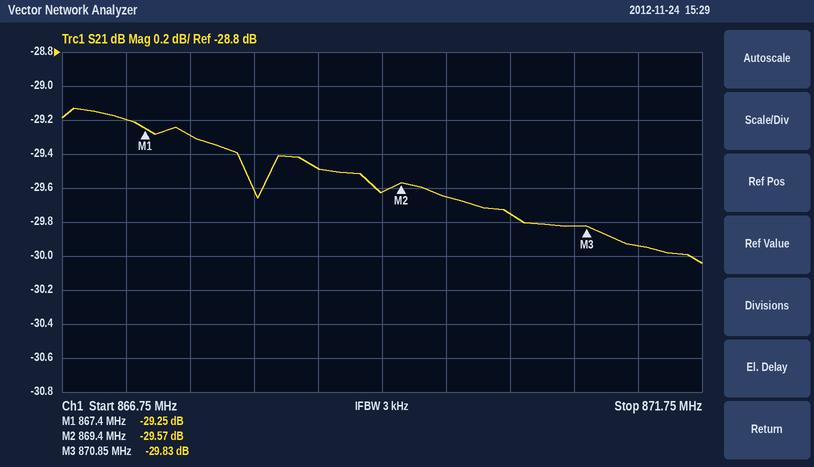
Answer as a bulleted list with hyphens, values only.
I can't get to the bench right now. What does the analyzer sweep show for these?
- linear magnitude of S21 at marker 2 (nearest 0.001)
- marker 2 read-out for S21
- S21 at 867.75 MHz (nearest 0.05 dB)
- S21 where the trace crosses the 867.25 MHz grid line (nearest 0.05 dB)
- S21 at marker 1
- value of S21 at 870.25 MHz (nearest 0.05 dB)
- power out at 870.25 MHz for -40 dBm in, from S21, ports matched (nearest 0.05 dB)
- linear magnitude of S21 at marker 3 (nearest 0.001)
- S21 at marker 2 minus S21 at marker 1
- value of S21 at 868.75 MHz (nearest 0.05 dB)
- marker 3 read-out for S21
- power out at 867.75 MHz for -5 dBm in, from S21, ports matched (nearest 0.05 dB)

- 0.033
- -29.57 dB
- -29.30 dB
- -29.20 dB
- -29.25 dB
- -29.75 dB
- -69.75 dBm
- 0.032
- -0.32 dB
- -29.50 dB
- -29.83 dB
- -34.30 dBm
